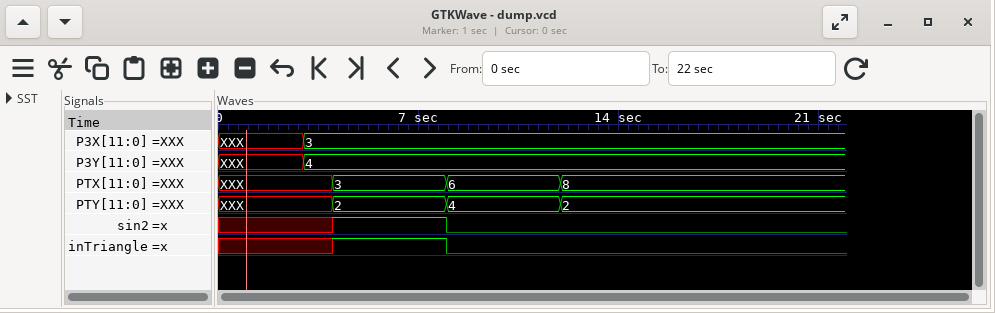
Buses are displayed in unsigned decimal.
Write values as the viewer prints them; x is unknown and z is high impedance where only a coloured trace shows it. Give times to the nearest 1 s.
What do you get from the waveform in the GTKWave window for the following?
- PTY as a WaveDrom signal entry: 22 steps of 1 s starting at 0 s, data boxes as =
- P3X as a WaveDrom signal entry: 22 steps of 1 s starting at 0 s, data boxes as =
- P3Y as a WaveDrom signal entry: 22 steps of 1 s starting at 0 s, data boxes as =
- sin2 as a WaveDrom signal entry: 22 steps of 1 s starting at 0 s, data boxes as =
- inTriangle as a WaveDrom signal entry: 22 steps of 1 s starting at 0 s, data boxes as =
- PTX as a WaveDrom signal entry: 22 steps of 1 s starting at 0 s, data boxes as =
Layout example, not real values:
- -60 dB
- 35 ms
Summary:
- {name: 'PTY', wave: 'x...=...=...=.........', data: '2 4 2'}
- {name: 'P3X', wave: 'x..=..................', data: '3'}
- {name: 'P3Y', wave: 'x..=..................', data: '4'}
- {name: 'sin2', wave: 'x...1...0.............'}
- {name: 'inTriangle', wave: 'x...1...0.............'}
- {name: 'PTX', wave: 'x...=...=...=.........', data: '3 6 8'}
